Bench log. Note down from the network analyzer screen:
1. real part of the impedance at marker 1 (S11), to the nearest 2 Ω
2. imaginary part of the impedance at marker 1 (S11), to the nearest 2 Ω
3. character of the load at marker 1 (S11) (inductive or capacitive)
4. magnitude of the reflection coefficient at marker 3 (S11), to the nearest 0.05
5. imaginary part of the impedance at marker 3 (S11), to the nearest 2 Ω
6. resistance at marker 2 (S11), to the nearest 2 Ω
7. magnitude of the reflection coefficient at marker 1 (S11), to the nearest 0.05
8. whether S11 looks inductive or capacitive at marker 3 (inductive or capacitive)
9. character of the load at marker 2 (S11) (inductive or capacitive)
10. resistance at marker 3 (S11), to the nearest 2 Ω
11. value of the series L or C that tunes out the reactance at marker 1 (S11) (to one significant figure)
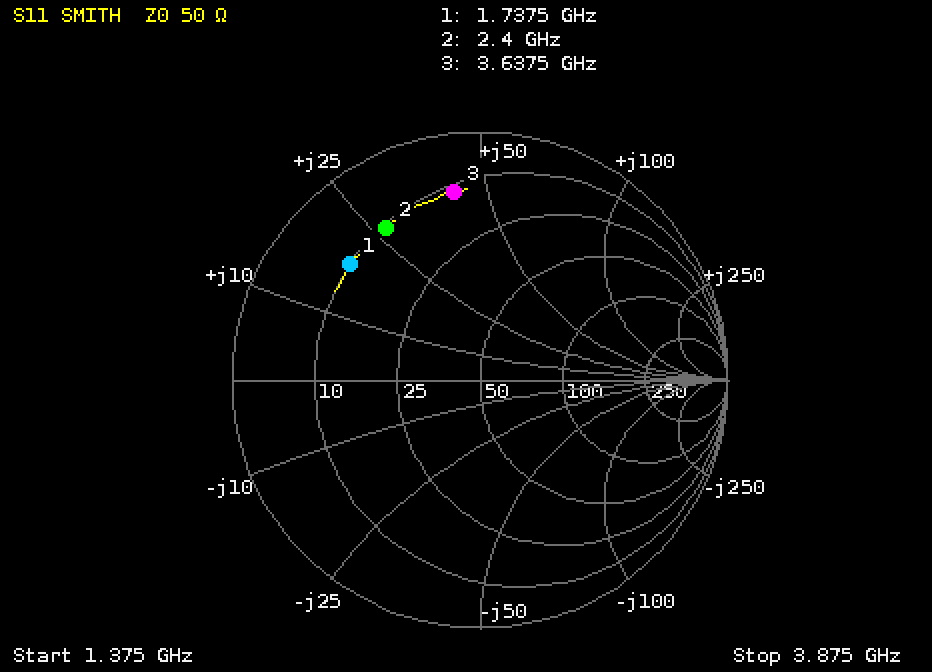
10 Ω
+18 Ω
inductive
0.75
+42 Ω
10 Ω
0.70
inductive
inductive
12 Ω
5 pF
